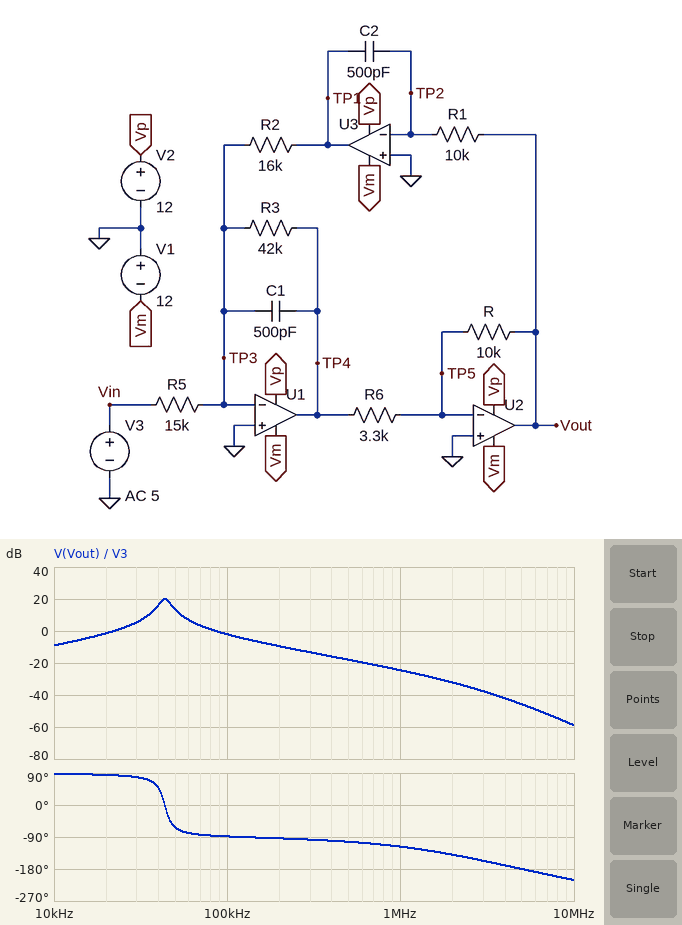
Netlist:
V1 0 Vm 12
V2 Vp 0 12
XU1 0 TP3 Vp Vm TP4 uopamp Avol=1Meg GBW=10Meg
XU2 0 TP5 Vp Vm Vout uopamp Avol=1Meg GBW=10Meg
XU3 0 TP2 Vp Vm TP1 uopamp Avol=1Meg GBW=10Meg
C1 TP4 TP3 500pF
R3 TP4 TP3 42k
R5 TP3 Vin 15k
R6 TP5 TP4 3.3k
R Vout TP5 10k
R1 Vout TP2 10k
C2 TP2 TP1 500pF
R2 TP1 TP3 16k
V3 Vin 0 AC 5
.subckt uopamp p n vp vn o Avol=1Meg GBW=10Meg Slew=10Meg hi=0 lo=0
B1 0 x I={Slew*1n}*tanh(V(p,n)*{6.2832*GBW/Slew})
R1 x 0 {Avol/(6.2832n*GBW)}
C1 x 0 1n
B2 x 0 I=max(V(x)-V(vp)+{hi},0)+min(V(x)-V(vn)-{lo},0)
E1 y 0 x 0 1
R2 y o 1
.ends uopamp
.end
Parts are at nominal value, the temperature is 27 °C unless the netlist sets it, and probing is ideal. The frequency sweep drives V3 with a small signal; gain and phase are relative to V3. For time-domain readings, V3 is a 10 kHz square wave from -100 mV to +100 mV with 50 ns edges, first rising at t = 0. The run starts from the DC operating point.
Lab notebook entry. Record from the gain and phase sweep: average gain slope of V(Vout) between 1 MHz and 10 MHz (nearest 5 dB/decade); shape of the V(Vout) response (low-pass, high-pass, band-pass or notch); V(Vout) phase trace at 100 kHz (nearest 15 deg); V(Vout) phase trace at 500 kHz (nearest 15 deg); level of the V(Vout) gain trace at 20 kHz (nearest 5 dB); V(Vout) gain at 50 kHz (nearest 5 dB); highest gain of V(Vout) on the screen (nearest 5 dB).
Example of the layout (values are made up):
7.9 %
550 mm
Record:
-35 dB/decade
band-pass
-90 deg
-105 deg
0 dB
15 dB
20 dB
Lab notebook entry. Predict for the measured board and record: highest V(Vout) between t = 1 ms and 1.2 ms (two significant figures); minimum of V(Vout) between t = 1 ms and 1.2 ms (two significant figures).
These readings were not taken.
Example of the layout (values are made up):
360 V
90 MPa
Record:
210 mV
-210 mV
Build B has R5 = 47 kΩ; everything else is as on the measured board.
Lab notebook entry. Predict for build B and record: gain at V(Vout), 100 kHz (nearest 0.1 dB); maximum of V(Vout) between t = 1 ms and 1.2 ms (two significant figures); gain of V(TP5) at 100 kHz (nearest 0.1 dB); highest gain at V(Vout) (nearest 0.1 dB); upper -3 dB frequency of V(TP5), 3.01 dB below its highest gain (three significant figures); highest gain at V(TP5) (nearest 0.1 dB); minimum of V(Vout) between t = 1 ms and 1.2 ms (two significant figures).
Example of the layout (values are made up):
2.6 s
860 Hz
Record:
-12.0 dB
68 mV
-52.0 dB
10.1 dB
47.6 kHz
-37.1 dB
-68 mV
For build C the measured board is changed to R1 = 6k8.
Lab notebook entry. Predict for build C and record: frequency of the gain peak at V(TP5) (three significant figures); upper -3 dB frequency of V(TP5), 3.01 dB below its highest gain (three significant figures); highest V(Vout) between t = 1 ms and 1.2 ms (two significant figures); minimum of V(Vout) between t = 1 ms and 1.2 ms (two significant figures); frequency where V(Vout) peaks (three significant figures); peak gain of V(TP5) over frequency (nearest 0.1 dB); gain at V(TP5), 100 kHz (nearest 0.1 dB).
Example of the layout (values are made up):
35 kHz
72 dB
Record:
53.0 kHz
56.3 kHz
280 mV
-280 mV
52.9 kHz
-24.8 dB
-41.1 dB
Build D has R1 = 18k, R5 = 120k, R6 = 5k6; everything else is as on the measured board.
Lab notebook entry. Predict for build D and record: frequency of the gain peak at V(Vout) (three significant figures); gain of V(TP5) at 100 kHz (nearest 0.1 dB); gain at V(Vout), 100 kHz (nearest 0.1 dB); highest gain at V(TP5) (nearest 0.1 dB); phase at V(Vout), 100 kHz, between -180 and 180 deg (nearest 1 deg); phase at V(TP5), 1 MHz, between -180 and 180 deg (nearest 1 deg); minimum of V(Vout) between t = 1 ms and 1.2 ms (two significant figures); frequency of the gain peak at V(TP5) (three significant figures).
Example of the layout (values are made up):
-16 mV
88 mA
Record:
25.0 kHz
-66.0 dB
-26.0 dB
-55.7 dB
-88 deg
159 deg
-27 mV
25.6 kHz
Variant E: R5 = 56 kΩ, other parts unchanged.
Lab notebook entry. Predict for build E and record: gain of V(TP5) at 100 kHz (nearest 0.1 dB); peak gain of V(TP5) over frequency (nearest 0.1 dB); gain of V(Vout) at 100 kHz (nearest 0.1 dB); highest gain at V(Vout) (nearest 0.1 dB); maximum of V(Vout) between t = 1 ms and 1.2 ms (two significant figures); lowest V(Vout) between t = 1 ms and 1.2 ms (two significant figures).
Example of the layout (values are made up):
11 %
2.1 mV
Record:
-53.5 dB
-38.6 dB
-13.5 dB
8.6 dB
57 mV
-57 mV
